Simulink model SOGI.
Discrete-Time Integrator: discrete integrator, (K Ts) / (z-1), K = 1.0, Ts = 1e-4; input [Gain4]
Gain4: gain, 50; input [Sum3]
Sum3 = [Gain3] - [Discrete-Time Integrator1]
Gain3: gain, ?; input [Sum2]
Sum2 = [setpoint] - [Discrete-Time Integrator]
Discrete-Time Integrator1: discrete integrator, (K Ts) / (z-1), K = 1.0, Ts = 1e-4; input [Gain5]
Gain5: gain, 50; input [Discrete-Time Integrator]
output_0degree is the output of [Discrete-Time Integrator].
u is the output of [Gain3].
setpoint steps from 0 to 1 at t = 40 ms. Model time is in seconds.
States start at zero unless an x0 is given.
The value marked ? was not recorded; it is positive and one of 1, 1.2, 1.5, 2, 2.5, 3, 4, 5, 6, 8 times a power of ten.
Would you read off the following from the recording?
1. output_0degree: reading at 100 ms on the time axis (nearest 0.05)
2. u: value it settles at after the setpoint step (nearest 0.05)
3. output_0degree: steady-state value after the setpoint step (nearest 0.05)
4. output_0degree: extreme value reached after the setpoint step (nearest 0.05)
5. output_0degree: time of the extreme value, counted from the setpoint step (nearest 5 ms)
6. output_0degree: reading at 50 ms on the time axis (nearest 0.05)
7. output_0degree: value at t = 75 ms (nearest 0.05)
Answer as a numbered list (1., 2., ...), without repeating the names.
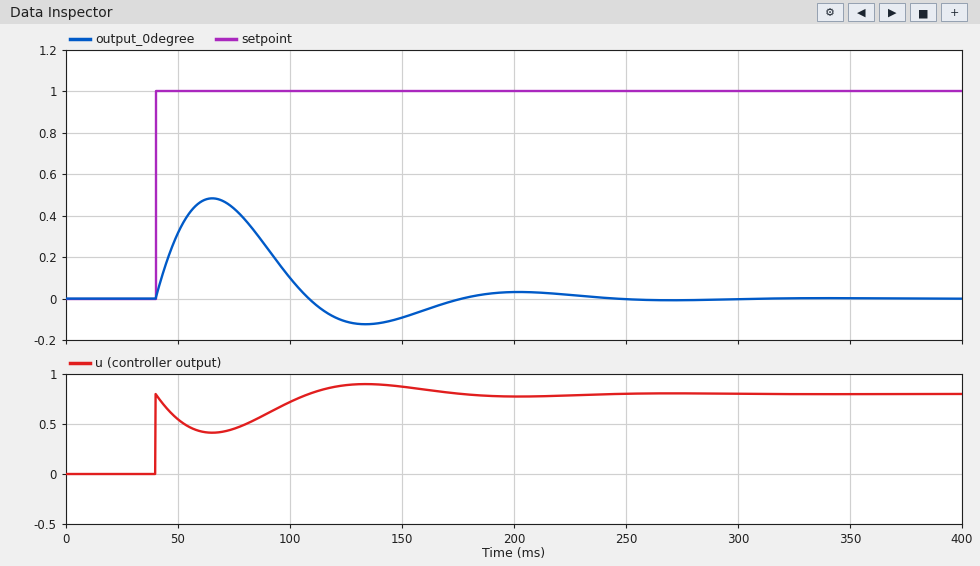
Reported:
1. 0.10
2. 0.80
3. 0.00
4. 0.50
5. 25 ms
6. 0.30
7. 0.45
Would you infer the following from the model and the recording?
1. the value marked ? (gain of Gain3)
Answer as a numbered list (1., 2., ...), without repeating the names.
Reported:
1. 0.8
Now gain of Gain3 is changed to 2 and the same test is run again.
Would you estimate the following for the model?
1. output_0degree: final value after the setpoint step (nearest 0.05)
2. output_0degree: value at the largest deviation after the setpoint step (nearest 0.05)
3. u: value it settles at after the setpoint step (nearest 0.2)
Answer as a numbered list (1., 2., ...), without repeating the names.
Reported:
1. 0.00
2. 0.75
3. 2.0
